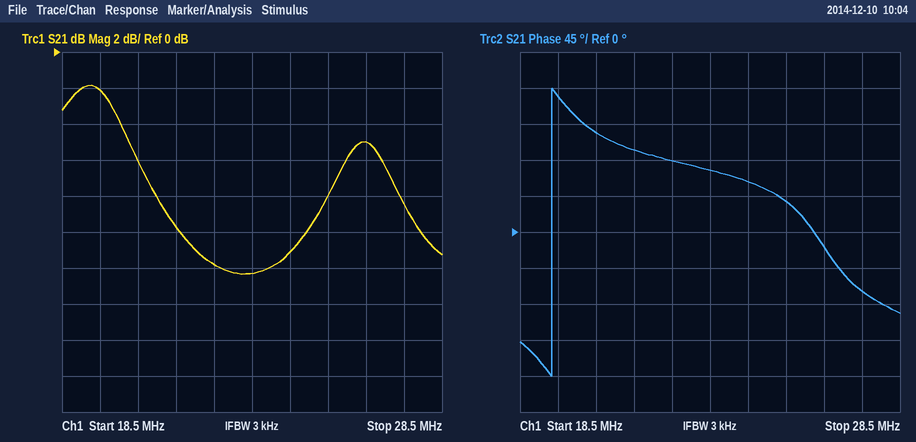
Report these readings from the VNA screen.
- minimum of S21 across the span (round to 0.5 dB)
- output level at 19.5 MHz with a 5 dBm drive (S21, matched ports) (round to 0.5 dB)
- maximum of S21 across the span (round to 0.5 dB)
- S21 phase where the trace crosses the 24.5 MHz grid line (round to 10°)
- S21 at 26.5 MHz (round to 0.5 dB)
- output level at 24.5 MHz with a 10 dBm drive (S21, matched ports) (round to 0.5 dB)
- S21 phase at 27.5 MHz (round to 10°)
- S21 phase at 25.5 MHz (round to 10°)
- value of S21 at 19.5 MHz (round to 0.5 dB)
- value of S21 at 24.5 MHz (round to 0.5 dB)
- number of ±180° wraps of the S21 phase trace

-12.5 dB
3.0 dBm
-2.0 dB
60°
-5.0 dB
-1.0 dBm
-70°
40°
-2.0 dB
-11.0 dB
1
